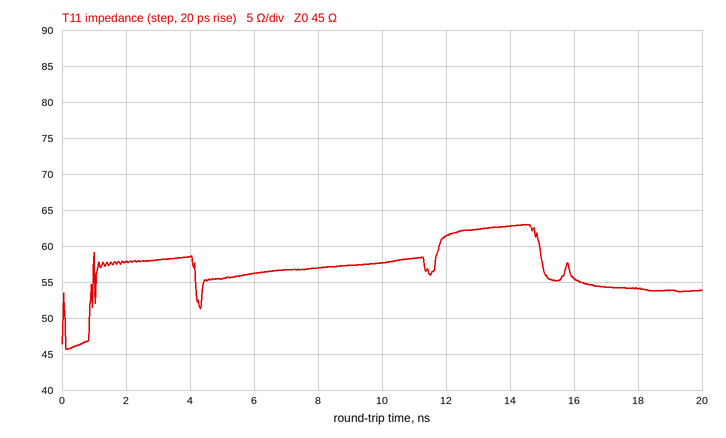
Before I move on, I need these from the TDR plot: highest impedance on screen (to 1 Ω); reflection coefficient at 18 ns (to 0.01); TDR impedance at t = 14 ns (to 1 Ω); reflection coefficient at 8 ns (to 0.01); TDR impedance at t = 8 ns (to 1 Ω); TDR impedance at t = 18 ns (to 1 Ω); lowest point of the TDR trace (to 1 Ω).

63 Ω
+0.09
63 Ω
+0.12
57 Ω
54 Ω
46 Ω
